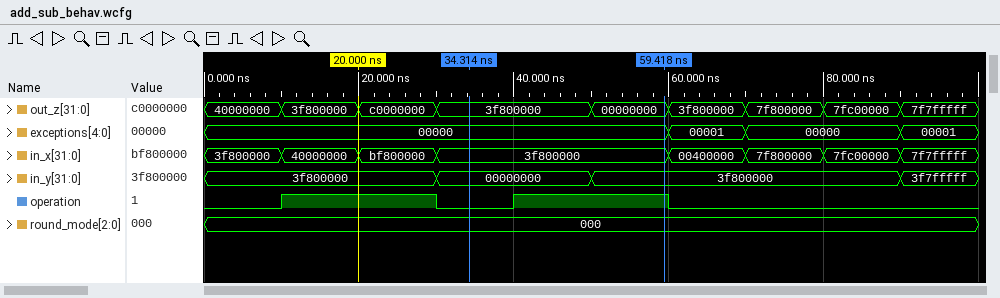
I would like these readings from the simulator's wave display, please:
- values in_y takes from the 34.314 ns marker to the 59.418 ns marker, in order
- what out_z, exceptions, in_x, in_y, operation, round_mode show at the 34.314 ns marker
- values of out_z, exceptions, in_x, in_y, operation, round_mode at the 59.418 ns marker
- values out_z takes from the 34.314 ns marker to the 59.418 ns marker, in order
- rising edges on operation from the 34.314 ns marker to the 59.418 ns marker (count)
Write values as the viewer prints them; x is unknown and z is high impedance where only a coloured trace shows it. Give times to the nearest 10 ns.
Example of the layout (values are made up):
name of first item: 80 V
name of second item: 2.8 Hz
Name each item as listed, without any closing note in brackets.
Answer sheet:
values in_y takes from the 34.314 ns marker to the 59.418 ns marker, in order: 00000000, 3f800000
what out_z, exceptions, in_x, in_y, operation, round_mode show at the 34.314 ns marker: out_z=3f800000, exceptions=00000, in_x=3f800000, in_y=00000000, operation=0, round_mode=000
values of out_z, exceptions, in_x, in_y, operation, round_mode at the 59.418 ns marker: out_z=00000000, exceptions=00000, in_x=3f800000, in_y=3f800000, operation=1, round_mode=000
values out_z takes from the 34.314 ns marker to the 59.418 ns marker, in order: 3f800000, 00000000
rising edges on operation from the 34.314 ns marker to the 59.418 ns marker: 1
